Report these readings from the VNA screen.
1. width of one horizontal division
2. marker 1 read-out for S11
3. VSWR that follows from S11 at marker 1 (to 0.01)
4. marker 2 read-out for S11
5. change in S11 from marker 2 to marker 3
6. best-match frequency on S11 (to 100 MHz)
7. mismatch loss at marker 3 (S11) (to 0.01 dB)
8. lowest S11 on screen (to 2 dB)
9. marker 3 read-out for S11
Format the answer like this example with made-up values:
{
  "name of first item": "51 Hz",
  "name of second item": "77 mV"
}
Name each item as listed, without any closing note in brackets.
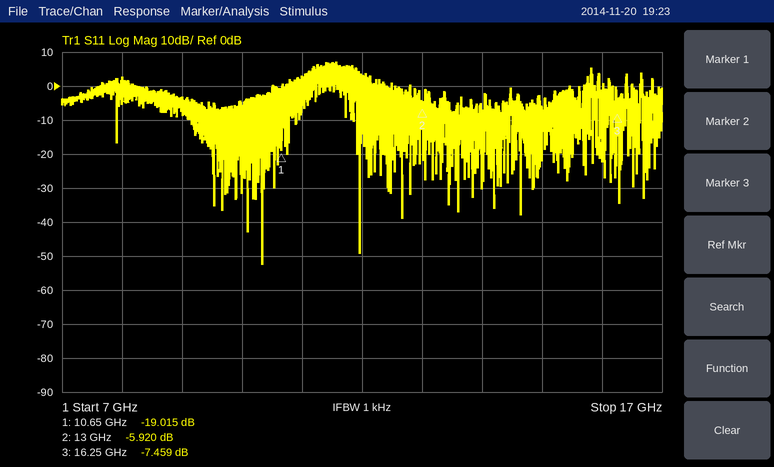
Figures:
{
  "width of one horizontal division": "1 GHz",
  "marker 1 read-out for S11": "-19.015 dB",
  "VSWR that follows from S11 at marker 1": "1.25",
  "marker 2 read-out for S11": "-5.920 dB",
  "change in S11 from marker 2 to marker 3": "-1.539 dB",
  "best-match frequency on S11": "10.3 GHz",
  "mismatch loss at marker 3 (S11)": "0.86 dB",
  "lowest S11 on screen": "-52 dB",
  "marker 3 read-out for S11": "-7.459 dB"
}
